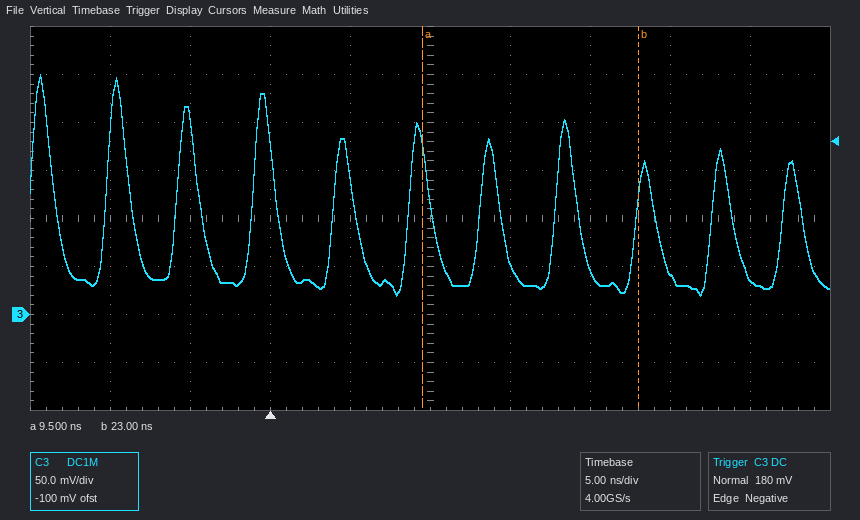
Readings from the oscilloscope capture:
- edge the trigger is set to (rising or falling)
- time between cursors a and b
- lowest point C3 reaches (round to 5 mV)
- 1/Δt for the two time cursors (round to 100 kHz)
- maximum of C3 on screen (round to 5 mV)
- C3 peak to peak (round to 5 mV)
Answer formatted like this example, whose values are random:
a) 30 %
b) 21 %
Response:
a) falling
b) 13.5 ns
c) 20 mV
d) 74.1 MHz
e) 250 mV
f) 230 mV
